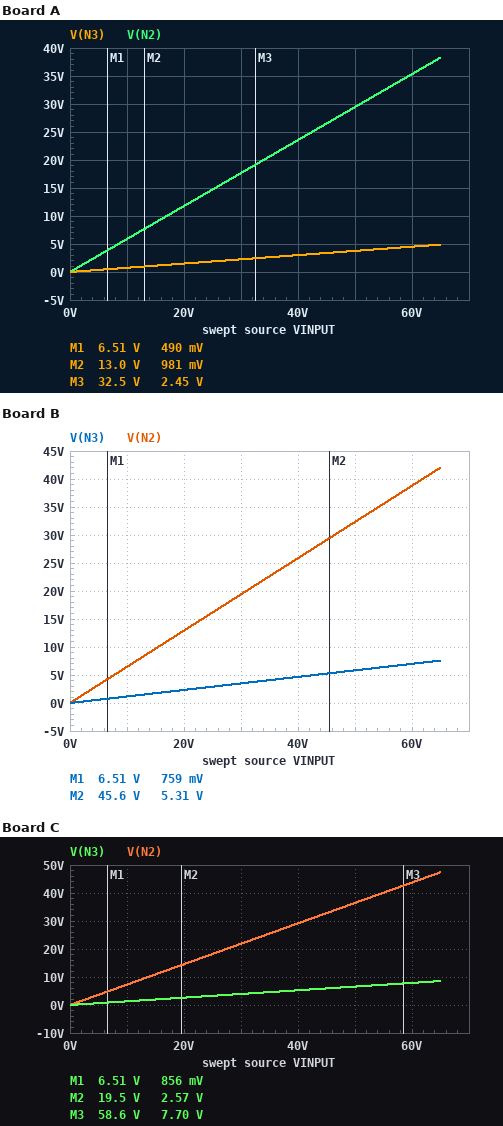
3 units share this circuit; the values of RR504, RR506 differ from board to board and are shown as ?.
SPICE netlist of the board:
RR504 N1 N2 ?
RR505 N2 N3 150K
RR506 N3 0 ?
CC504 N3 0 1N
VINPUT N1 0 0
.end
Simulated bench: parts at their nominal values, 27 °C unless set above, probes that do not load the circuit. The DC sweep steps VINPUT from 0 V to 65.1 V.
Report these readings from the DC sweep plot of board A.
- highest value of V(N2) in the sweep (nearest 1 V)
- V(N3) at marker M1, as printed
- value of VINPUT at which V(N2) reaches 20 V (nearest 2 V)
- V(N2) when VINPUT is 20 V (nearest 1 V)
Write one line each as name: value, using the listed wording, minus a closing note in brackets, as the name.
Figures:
highest value of V(N2) in the sweep: 38 V
V(N3) at marker M1, as printed: 490 mV
value of VINPUT at which V(N2) reaches 20 V: 34 V
V(N2) when VINPUT is 20 V: 12 V
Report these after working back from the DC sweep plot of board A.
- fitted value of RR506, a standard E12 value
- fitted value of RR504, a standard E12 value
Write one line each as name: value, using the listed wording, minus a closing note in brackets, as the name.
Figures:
fitted value of RR506, a standard E12 value: 22 kΩ
fitted value of RR504, a standard E12 value: 120 kΩ
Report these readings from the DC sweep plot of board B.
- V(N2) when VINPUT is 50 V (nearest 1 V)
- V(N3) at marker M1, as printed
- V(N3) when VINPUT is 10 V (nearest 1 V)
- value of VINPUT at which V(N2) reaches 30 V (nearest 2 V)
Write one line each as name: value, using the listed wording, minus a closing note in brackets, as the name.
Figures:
V(N2) when VINPUT is 50 V: 32 V
V(N3) at marker M1, as printed: 759 mV
V(N3) when VINPUT is 10 V: 1 V
value of VINPUT at which V(N2) reaches 30 V: 46 V
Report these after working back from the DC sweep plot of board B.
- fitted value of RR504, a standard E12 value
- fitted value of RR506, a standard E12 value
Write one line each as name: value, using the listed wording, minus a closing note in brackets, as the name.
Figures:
fitted value of RR504, a standard E12 value: 100 kΩ
fitted value of RR506, a standard E12 value: 33 kΩ
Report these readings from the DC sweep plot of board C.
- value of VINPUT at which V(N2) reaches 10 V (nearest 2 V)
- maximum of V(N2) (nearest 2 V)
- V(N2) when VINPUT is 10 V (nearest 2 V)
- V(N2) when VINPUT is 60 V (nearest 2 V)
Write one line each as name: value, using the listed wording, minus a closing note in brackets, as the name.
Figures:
value of VINPUT at which V(N2) reaches 10 V: 14 V
maximum of V(N2): 48 V
V(N2) when VINPUT is 10 V: 8 V
V(N2) when VINPUT is 60 V: 44 V
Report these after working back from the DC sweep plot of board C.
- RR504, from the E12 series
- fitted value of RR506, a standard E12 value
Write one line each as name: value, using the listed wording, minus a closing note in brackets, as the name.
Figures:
RR504, from the E12 series: 68 kΩ
fitted value of RR506, a standard E12 value: 33 kΩ
